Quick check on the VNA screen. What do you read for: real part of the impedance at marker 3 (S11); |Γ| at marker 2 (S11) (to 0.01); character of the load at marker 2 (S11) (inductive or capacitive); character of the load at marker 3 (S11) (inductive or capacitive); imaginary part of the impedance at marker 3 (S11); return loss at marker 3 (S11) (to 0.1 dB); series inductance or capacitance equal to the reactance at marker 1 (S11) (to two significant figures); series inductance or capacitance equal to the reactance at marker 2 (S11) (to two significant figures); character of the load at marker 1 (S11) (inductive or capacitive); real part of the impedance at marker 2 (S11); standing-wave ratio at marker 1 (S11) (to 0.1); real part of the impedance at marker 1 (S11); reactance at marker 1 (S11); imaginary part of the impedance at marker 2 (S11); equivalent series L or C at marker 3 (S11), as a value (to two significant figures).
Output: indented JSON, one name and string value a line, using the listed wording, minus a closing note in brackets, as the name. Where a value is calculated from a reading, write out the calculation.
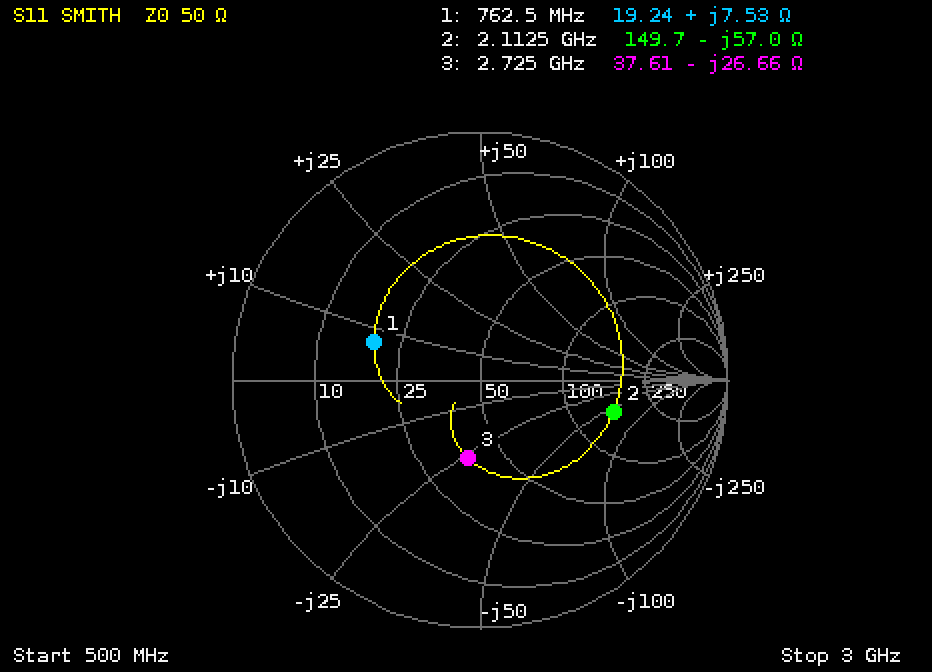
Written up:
{
  "real part of the impedance at marker 3": "37.61 Ω",
  "|Γ| at marker 2 (S11)": "0.55",
  "character of the load at marker 2 (S11)": "capacitive",
  "character of the load at marker 3 (S11)": "capacitive",
  "imaginary part of the impedance at marker 3": "-26.66 Ω",
  "return loss at marker 3 (S11)": "9.9 dB",
  "series inductance or capacitance equal to the reactance at marker 1 (S11)": "L = 7.53 Ω/(2π × 762.5 MHz) ≈ 1.6 nH",
  "series inductance or capacitance equal to the reactance at marker 2 (S11)": "C = 1/(2π × 2.1125 GHz × 57 Ω) ≈ 1.3 pF",
  "character of the load at marker 1 (S11)": "inductive",
  "real part of the impedance at marker 2": "149.7 Ω",
  "standing-wave ratio at marker 1 (S11)": "2.7",
  "real part of the impedance at marker 1": "19.24 Ω",
  "reactance at marker 1": "+7.53 Ω",
  "imaginary part of the impedance at marker 2": "-57.0 Ω",
  "equivalent series L or C at marker 3 (S11), as a value": "C = 1/(2π × 2.725 GHz × 26.66 Ω) ≈ 2.2 pF"
}
